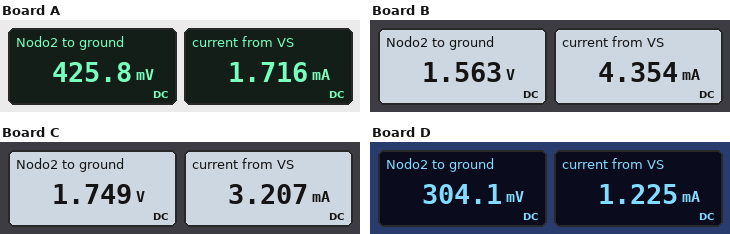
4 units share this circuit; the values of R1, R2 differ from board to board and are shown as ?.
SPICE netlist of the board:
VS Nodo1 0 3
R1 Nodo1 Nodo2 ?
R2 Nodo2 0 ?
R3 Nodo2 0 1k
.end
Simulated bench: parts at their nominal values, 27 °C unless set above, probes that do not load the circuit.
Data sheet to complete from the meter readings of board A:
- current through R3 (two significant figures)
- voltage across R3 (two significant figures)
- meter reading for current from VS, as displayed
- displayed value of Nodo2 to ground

430 µA
430 mV
1.716 mA
425.8 mV
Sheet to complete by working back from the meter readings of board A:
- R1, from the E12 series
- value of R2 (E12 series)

1.5 kΩ
330 Ω
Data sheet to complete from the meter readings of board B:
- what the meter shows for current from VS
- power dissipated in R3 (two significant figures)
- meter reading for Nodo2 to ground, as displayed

4.354 mA
2.4 mW
1.563 V
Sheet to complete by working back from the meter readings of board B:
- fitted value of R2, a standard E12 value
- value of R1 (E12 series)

560 Ω
330 Ω
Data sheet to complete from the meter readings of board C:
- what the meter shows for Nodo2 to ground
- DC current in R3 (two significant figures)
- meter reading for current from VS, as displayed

1.749 V
1.7 mA
3.207 mA
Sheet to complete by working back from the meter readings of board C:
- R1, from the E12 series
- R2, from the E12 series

390 Ω
1.2 kΩ
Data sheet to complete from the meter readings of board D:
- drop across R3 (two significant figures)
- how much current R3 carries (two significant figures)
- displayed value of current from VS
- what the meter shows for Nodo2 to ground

300 mV
300 µA
1.225 mA
304.1 mV
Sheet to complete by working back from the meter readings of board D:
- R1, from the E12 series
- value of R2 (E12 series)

2.2 kΩ
330 Ω
